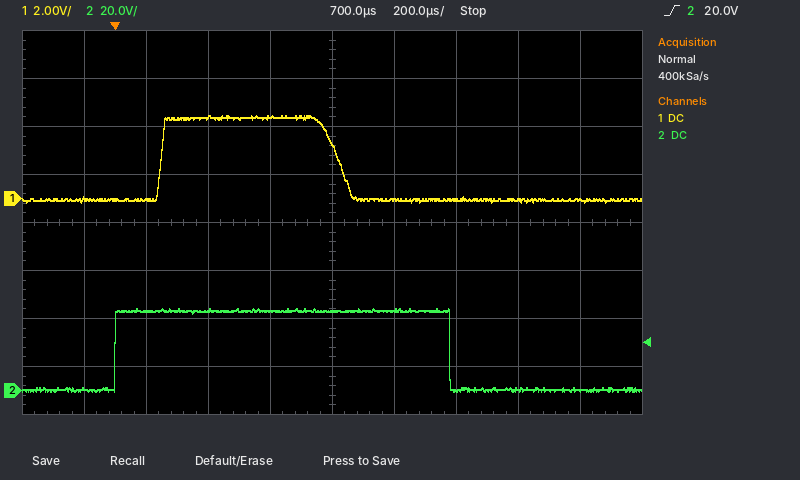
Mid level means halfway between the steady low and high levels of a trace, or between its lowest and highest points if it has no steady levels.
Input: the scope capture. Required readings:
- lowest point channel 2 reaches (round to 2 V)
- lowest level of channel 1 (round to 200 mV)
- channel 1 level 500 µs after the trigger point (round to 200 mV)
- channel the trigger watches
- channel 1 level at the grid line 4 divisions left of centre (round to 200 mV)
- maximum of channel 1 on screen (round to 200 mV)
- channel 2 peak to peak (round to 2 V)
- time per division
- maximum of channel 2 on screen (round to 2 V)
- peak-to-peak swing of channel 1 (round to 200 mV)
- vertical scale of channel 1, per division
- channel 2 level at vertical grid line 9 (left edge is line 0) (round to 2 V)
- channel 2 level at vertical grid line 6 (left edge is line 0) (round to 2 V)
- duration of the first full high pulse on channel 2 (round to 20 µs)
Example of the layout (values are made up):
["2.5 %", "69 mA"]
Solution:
["0 V", "-200 mV", "3.4 V", "channel 2", "0.0 V", "3.4 V", "34 V", "200 µs", "34 V", "3.6 V", "2 V", "0 V", "34 V", "1.08 ms"]
